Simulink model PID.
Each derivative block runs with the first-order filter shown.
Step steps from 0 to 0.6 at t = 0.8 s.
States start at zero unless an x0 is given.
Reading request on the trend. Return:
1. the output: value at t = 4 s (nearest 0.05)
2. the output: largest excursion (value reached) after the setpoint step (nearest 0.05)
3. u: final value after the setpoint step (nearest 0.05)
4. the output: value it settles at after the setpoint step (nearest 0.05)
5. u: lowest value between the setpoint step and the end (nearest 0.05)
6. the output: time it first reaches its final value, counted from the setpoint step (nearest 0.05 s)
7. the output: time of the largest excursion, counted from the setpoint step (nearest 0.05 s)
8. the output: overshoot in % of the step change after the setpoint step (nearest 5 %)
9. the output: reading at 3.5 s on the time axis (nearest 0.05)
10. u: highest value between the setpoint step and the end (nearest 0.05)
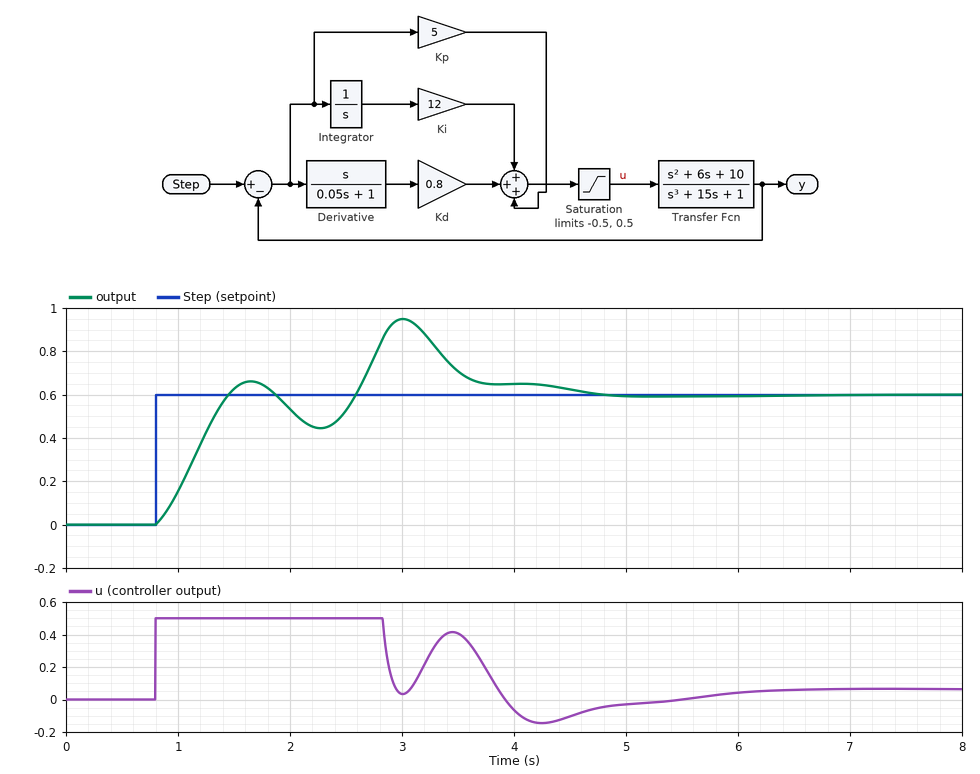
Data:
0.65
0.95
0.05
0.60
-0.15
0.65 s
2.20 s
60 %
0.70
0.50
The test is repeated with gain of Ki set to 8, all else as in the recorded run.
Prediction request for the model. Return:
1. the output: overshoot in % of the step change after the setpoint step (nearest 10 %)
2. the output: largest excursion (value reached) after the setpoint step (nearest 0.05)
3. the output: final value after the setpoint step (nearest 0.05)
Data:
40 %
0.85
0.60
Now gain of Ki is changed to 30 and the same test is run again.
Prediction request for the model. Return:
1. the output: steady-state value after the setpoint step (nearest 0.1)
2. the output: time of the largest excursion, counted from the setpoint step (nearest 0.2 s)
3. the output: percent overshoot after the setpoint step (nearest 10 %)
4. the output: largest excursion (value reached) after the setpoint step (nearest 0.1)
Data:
0.6
2.4 s
80 %
1.1
